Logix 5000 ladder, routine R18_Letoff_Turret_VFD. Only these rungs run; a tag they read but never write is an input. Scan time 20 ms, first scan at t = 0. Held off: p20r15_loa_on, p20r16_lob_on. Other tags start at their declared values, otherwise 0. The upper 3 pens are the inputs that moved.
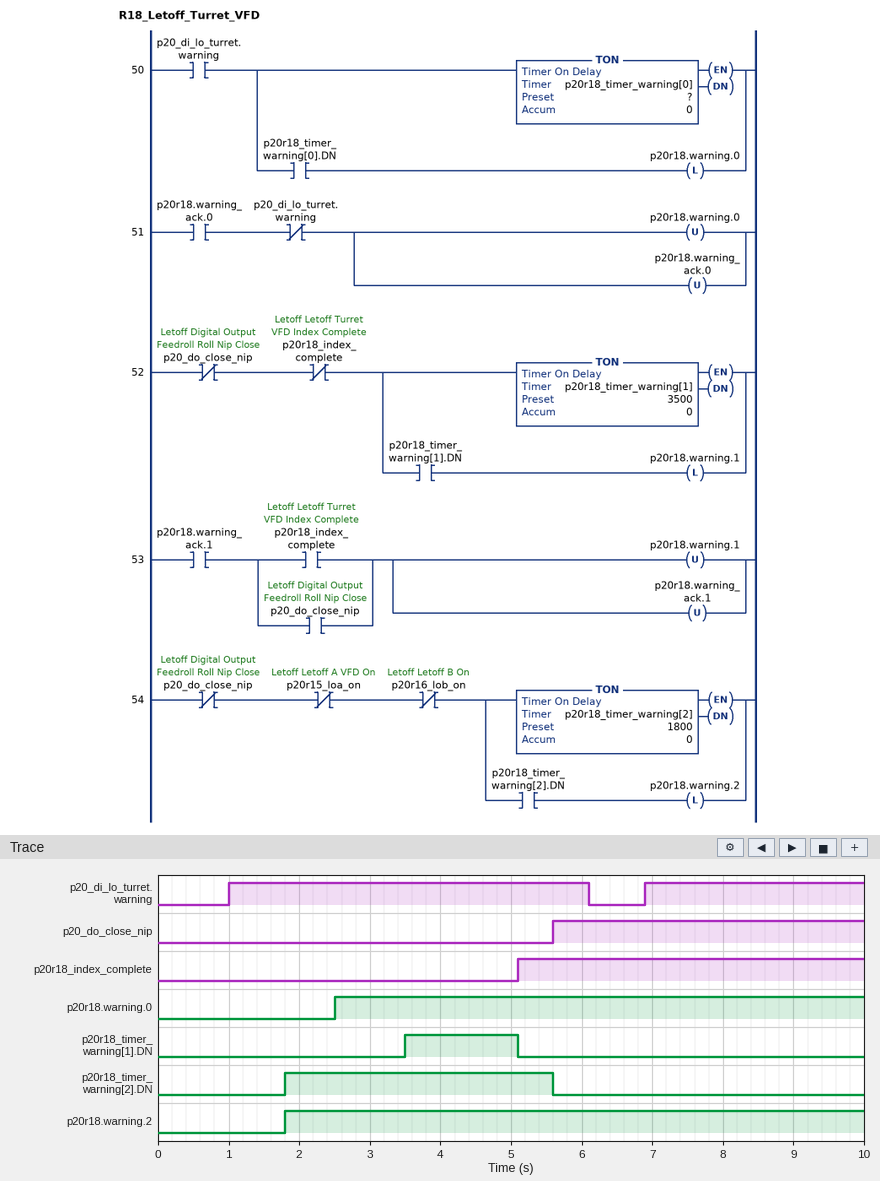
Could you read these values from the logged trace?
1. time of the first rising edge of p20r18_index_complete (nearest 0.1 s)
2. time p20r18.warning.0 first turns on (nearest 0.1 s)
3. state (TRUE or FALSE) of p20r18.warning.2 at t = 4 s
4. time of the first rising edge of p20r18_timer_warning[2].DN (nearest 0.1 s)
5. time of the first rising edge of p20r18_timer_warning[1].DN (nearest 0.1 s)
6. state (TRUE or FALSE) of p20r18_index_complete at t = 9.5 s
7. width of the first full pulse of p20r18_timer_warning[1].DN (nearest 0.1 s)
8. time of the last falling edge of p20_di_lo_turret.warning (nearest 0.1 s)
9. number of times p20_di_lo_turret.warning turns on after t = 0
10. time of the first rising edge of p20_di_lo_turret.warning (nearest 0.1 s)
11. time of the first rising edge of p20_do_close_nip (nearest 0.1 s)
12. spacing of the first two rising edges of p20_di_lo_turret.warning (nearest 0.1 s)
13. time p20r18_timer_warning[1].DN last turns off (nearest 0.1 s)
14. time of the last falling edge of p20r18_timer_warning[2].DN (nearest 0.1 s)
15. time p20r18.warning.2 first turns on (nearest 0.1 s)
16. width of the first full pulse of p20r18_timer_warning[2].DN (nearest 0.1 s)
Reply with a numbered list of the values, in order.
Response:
1. 5.1 s
2. 2.5 s
3. TRUE
4. 1.8 s
5. 3.5 s
6. TRUE
7. 1.6 s
8. 6.1 s
9. 2
10. 1.0 s
11. 5.6 s
12. 5.9 s
13. 5.1 s
14. 5.6 s
15. 1.8 s
16. 3.8 s
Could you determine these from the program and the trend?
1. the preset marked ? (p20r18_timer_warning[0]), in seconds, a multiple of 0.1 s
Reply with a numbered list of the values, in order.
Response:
1. 1.5 s
